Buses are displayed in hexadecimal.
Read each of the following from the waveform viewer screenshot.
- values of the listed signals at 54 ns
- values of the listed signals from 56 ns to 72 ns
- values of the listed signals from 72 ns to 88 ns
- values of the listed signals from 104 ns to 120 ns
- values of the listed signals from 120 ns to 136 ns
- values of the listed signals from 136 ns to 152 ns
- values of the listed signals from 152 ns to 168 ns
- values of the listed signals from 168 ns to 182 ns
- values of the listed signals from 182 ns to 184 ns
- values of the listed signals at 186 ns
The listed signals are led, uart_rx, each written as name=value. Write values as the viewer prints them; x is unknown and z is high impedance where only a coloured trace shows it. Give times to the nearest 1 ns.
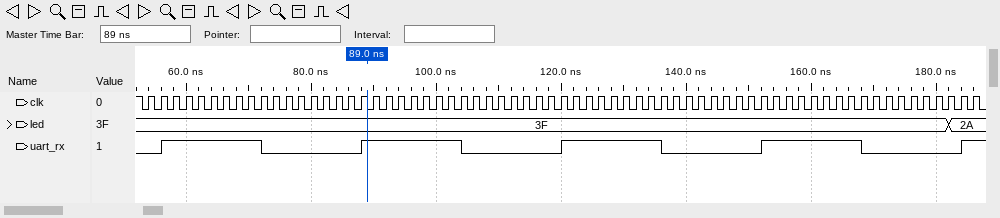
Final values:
led=3F, uart_rx=0
led=3F, uart_rx=1
led=3F, uart_rx=0
led=3F, uart_rx=0
led=3F, uart_rx=1
led=3F, uart_rx=0
led=3F, uart_rx=1
led=3F, uart_rx=0
led=2A, uart_rx=0
led=2A, uart_rx=1
